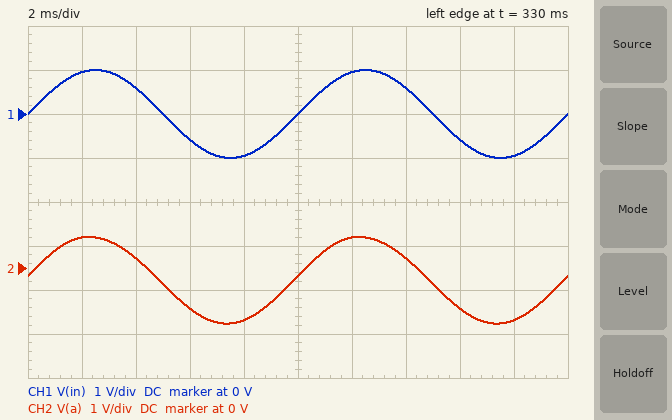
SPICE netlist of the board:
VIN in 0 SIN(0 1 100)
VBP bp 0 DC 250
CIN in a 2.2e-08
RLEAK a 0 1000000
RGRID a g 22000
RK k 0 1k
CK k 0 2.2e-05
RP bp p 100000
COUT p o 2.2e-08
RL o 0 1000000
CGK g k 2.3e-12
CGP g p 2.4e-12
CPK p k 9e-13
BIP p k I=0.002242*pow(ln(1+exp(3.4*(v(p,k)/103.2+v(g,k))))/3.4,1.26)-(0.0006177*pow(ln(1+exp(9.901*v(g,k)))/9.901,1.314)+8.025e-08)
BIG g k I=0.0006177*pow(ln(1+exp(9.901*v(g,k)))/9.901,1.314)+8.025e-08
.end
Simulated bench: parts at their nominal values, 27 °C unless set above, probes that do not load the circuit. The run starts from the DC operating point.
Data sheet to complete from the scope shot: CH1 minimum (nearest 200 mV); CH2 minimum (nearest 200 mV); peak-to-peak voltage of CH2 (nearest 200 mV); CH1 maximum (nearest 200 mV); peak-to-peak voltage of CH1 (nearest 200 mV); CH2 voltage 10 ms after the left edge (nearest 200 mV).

-1.0 V
-1.2 V
2.0 V
1.0 V
2.0 V
-200 mV
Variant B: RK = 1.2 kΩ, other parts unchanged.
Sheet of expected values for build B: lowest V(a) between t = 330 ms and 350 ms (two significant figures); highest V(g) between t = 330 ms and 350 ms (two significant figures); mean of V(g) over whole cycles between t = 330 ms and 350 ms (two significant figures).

-1.2 V
770 mV
-200 mV
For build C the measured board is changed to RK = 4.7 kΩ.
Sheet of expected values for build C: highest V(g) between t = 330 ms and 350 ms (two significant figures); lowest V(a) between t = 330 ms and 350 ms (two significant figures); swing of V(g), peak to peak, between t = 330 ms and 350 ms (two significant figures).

910 mV
-1.1 V
2.0 V
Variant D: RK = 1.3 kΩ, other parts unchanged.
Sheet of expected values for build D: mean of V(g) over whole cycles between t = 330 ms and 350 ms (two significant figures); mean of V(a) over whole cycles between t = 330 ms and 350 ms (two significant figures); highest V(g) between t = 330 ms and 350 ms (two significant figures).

-170 mV
-160 mV
810 mV
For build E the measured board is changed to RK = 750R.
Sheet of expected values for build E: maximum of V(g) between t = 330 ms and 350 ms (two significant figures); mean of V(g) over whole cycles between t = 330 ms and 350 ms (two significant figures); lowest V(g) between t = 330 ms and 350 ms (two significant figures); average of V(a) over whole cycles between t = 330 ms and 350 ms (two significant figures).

510 mV
-420 mV
-1.4 V
-410 mV
